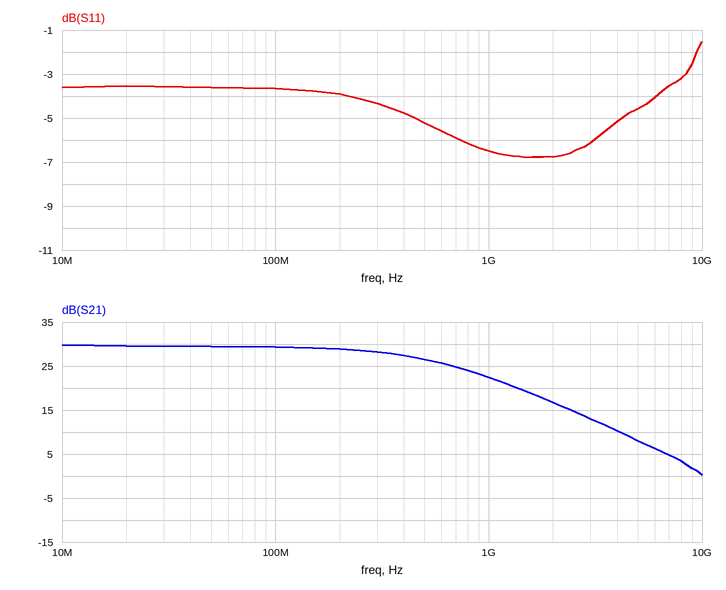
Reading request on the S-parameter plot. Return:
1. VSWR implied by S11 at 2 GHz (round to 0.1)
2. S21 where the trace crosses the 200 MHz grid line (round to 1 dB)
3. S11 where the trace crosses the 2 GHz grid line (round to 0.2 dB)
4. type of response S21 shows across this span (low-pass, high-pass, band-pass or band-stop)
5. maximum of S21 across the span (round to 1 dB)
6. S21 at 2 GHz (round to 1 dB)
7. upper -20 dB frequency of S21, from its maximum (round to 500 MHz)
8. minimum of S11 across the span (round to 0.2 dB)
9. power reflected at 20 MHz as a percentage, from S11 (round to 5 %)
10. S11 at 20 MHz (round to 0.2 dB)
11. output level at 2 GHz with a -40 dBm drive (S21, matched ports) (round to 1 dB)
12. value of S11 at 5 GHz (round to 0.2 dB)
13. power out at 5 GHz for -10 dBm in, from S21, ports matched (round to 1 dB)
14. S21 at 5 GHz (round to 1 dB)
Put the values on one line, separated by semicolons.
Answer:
2.7; 29 dB; -6.8 dB; low-pass; 30 dB; 17 dB; 4.0 GHz; -6.8 dB; 45 %; -3.6 dB; -23 dBm; -4.6 dB; -2 dBm; 8 dB
